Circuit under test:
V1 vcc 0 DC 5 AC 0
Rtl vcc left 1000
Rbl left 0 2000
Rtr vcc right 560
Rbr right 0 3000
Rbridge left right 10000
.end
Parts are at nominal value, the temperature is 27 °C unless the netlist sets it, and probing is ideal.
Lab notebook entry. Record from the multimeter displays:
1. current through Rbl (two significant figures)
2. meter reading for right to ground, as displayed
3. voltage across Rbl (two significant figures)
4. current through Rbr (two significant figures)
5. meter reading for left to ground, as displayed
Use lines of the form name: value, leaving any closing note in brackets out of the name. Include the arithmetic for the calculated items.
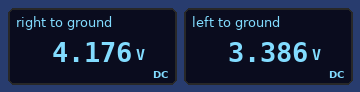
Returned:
current through Rbl: (3.386 V) / 2 kΩ = 1.7 mA
meter reading for right to ground, as displayed: 4.176 V
voltage across Rbl: 3.386 V = 3.4 V
current through Rbr: (4.176 V) / 3 kΩ = 1.4 mA
meter reading for left to ground, as displayed: 3.386 V
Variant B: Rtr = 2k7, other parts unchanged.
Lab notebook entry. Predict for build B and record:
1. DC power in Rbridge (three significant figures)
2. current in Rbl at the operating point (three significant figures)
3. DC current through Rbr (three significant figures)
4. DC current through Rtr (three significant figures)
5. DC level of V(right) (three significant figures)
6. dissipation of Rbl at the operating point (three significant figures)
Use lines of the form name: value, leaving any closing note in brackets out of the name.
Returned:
DC power in Rbridge: 33.7 µW
current in Rbl at the operating point: 1.65 mA
DC current through Rbr: 905 µA
DC current through Rtr: 847 µA
DC level of V(right): 2.71 V
dissipation of Rbl at the operating point: 5.43 mW
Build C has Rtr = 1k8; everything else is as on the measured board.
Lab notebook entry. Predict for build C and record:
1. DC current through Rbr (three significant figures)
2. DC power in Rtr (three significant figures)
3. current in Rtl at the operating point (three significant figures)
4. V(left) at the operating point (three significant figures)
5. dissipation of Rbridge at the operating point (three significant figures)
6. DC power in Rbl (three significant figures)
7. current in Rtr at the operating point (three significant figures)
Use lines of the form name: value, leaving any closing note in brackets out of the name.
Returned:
DC current through Rbr: 1.05 mA
DC power in Rtr: 1.91 mW
current in Rtl at the operating point: 1.68 mA
V(left) at the operating point: 3.32 V
dissipation of Rbridge at the operating point: 3.12 µW
DC power in Rbl: 5.52 mW
current in Rtr at the operating point: 1.03 mA
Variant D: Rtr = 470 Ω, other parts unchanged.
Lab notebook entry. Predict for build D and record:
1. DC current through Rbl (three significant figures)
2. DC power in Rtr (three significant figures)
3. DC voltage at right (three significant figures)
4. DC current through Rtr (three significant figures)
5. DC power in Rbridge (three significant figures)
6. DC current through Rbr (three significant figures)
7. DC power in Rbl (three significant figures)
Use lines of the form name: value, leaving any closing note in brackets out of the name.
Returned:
DC current through Rbl: 1.70 mA
DC power in Rtr: 1.08 mW
DC voltage at right: 4.29 V
DC current through Rtr: 1.52 mA
DC power in Rbridge: 79.8 µW
DC current through Rbr: 1.43 mA
DC power in Rbl: 5.76 mW
